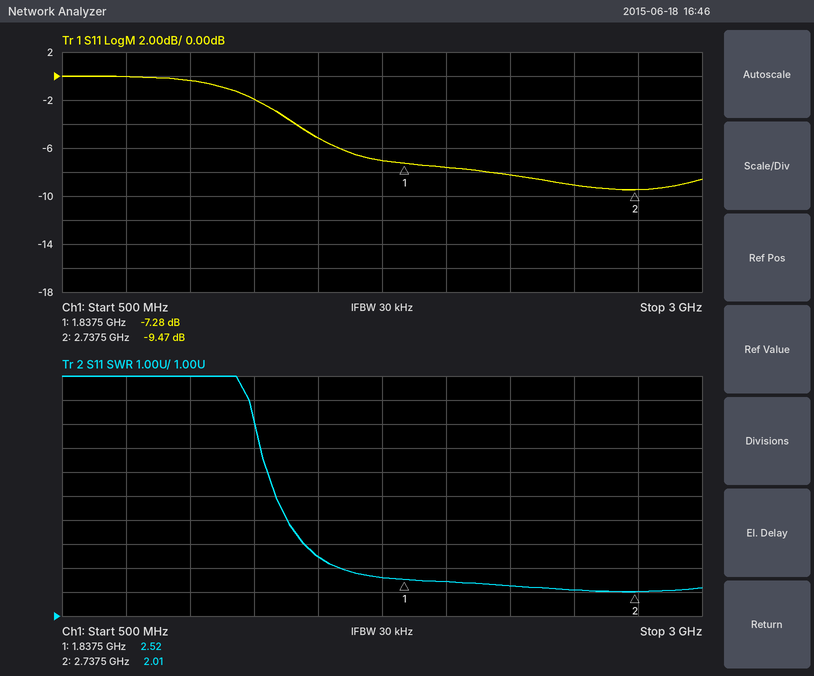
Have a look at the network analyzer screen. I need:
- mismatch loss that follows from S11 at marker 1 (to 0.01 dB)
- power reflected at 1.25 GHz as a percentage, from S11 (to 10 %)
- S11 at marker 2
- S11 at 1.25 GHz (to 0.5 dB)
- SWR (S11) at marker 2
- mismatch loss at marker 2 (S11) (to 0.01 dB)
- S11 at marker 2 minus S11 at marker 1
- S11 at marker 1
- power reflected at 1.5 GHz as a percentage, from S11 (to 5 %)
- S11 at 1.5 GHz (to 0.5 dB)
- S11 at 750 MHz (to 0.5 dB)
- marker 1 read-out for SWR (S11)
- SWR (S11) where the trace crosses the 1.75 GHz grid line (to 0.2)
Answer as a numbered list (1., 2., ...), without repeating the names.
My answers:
1. 0.90 dB
2. 60 %
3. -9.47 dB
4. -2.0 dB
5. 2.01
6. 0.52 dB
7. -2.19 dB
8. -7.28 dB
9. 30 %
10. -5.0 dB
11. 0.0 dB
12. 2.52
13. 2.6
